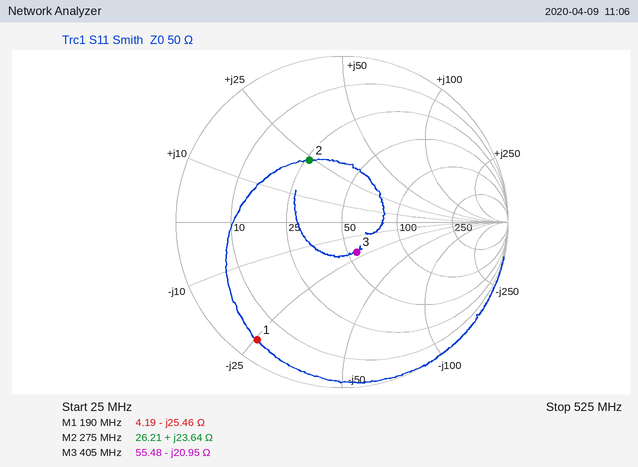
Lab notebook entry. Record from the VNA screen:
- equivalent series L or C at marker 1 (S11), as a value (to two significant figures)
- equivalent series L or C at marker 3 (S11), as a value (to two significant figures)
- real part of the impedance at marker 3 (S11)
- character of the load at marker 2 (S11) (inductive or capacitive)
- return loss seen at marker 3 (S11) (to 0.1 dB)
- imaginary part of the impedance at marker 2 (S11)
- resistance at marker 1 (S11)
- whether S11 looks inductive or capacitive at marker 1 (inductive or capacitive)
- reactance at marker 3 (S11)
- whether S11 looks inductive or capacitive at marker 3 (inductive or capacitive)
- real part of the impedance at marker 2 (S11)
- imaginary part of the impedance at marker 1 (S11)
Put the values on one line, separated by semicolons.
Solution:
33 pF; 19 pF; 55.48 Ω; inductive; 13.9 dB; +23.64 Ω; 4.19 Ω; capacitive; -20.95 Ω; capacitive; 26.21 Ω; -25.46 Ω
